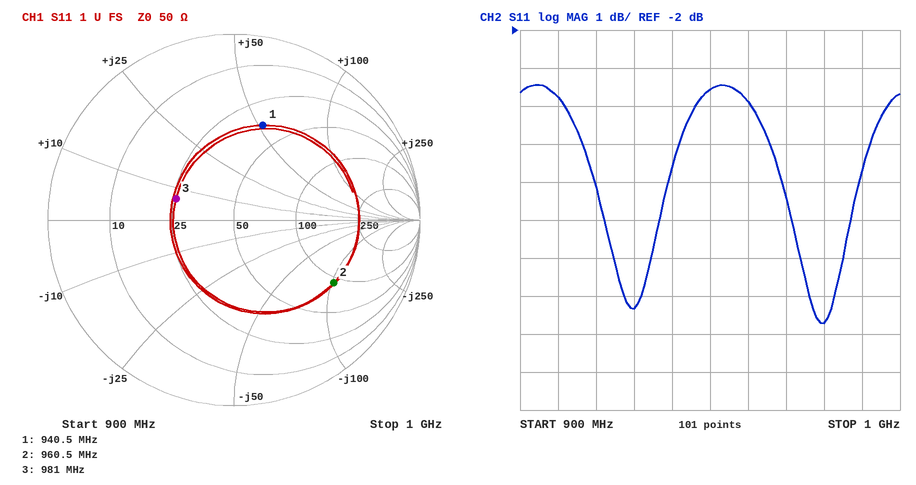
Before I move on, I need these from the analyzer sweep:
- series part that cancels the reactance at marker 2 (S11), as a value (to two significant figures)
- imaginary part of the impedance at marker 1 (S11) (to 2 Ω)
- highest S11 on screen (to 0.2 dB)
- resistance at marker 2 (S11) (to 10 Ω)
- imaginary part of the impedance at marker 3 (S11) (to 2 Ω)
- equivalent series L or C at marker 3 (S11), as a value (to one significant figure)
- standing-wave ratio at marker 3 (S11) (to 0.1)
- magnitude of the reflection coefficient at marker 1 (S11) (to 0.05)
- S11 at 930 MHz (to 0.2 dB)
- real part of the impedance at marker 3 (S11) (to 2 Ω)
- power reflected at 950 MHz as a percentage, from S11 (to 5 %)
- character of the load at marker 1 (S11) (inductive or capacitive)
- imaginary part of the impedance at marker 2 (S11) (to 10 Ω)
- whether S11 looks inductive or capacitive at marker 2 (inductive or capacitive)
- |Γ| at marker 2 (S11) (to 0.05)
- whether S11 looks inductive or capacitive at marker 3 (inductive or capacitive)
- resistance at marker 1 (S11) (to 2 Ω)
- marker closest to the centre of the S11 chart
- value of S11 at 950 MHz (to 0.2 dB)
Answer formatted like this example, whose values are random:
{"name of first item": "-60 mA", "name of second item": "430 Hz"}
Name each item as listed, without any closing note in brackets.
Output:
{"series part that cancels the reactance at marker 2 (S11), as a value": "17 nH", "imaginary part of the impedance at marker 1 (S11)": "+52 Ω", "highest S11 on screen": "-3.4 dB", "resistance at marker 2 (S11)": "90 Ω", "imaginary part of the impedance at marker 3 (S11)": "+6 Ω", "equivalent series L or C at marker 3 (S11), as a value": "1 nH", "standing-wave ratio at marker 3 (S11)": "2.0", "magnitude of the reflection coefficient at marker 1 (S11)": "0.55", "S11 at 930 MHz": "-9.4 dB", "real part of the impedance at marker 3 (S11)": "26 Ω", "power reflected at 950 MHz as a percentage, from S11": "45 %", "character of the load at marker 1 (S11)": "inductive", "imaginary part of the impedance at marker 2 (S11)": "-100 Ω", "whether S11 looks inductive or capacitive at marker 2": "capacitive", "|Γ| at marker 2 (S11)": "0.65", "whether S11 looks inductive or capacitive at marker 3": "inductive", "resistance at marker 1 (S11)": "36 Ω", "marker closest to the centre of the S11 chart": "marker 3", "value of S11 at 950 MHz": "-3.6 dB"}
